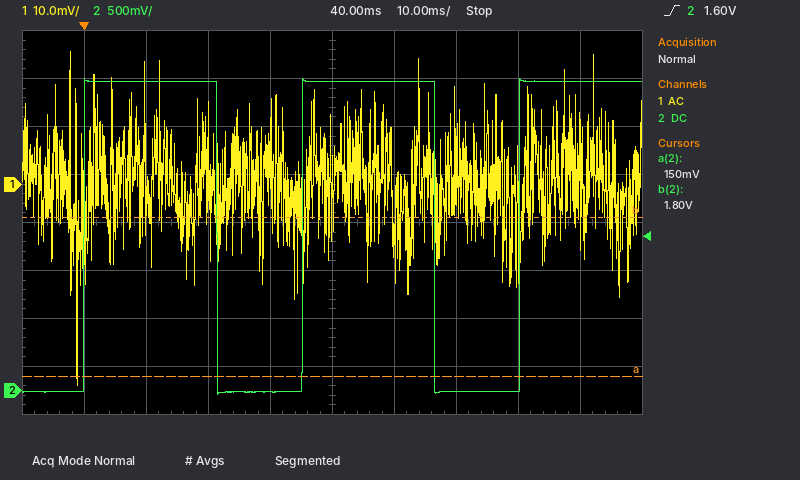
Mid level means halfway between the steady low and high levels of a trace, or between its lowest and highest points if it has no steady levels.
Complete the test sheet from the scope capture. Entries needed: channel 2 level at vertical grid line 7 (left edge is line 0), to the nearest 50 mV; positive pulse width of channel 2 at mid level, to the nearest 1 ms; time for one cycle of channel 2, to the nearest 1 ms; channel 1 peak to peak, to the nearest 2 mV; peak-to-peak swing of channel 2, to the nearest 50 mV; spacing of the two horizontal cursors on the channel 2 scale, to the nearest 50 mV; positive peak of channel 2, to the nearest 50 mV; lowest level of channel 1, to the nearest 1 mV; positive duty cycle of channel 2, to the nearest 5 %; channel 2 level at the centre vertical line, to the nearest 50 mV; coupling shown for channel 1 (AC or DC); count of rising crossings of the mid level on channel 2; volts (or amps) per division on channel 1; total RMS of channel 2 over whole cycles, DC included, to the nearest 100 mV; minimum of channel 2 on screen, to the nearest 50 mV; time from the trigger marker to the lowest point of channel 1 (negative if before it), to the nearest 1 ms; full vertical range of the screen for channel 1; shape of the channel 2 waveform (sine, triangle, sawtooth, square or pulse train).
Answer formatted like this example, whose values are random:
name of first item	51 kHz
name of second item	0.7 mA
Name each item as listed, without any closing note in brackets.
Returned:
channel 2 level at vertical grid line 7 (left edge is line 0), to the nearest 50 mV	0 mV
positive pulse width of channel 2 at mid level, to the nearest 1 ms	21 ms
time for one cycle of channel 2, to the nearest 1 ms	35 ms
channel 1 peak to peak, to the nearest 2 mV	70 mV
peak-to-peak swing of channel 2, to the nearest 50 mV	3.30 V
spacing of the two horizontal cursors on the channel 2 scale, to the nearest 50 mV	1.65 V
positive peak of channel 2, to the nearest 50 mV	3.25 V
lowest level of channel 1, to the nearest 1 mV	-42 mV
positive duty cycle of channel 2, to the nearest 5 %	60 %
channel 2 level at the centre vertical line, to the nearest 50 mV	3.20 V
coupling shown for channel 1	AC
count of rising crossings of the mid level on channel 2	3
volts (or amps) per division on channel 1	10 mV
total RMS of channel 2 over whole cycles, DC included, to the nearest 100 mV	2.5 V
minimum of channel 2 on screen, to the nearest 50 mV	-50 mV
time from the trigger marker to the lowest point of channel 1 (negative if before it), to the nearest 1 ms	-1 ms
full vertical range of the screen for channel 1	80 mV
shape of the channel 2 waveform	pulse train
